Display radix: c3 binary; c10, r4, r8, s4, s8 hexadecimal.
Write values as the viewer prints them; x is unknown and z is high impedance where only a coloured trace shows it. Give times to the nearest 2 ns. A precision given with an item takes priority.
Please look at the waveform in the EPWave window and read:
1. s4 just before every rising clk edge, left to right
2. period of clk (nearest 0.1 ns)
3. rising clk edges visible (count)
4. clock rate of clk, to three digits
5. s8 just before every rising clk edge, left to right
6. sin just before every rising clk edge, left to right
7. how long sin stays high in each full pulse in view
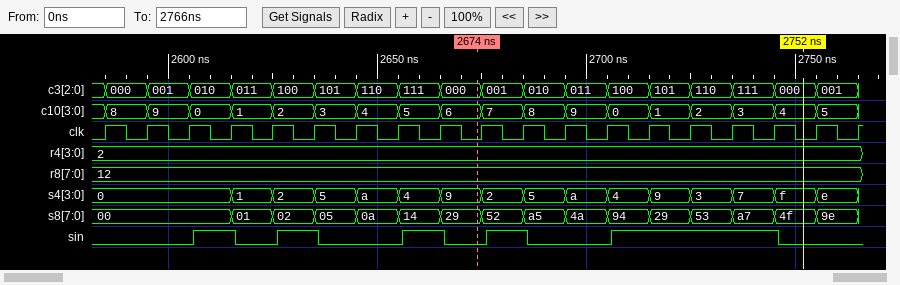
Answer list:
0, 0, 0, 0, 1, 2, 5, a, 4, 9, 2, 5, a, 4, 9, 3, 7, f, e
10 ns
19
100 MHz
00, 00, 00, 00, 01, 02, 05, 0a, 14, 29, 52, a5, 4a, 94, 29, 53, a7, 4f, 9e
0 0 0 1 0 1 0 0 1 0 1 0 0 1 1 1 1 0 0
10 ns, 10 ns, 10 ns, 10 ns, 40 ns
